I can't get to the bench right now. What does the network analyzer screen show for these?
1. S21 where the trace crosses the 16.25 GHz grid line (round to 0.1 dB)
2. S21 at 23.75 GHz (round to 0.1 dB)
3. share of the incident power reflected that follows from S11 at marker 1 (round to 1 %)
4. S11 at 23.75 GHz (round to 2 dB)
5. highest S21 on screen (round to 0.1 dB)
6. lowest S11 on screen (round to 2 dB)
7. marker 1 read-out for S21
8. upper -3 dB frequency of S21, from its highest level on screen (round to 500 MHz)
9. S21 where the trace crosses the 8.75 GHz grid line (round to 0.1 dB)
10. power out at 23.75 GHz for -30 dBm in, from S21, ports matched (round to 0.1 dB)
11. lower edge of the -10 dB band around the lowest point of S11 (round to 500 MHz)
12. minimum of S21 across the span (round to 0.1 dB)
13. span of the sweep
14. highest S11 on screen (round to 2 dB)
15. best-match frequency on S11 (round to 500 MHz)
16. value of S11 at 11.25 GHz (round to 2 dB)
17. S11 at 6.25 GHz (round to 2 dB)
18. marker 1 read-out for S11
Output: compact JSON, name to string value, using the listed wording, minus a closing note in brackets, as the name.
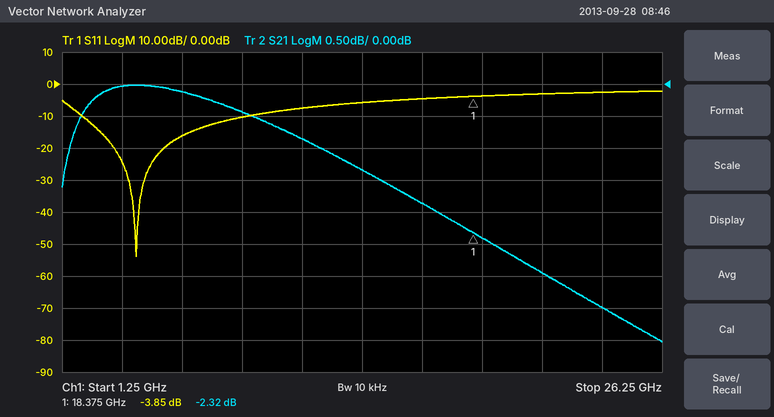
{"S21 where the trace crosses the 16.25 GHz grid line": "-1.9 dB", "S21 at 23.75 GHz": "-3.5 dB", "share of the incident power reflected that follows from S11 at marker 1": "41 %", "S11 at 23.75 GHz": "-2 dB", "highest S21 on screen": "0.0 dB", "lowest S11 on screen": "-54 dB", "marker 1 read-out for S21": "-2.32 dB", "upper -3 dB frequency of S21, from its highest level on screen": "21.5 GHz", "S21 where the trace crosses the 8.75 GHz grid line": "-0.4 dB", "power out at 23.75 GHz for -30 dBm in, from S21, ports matched": "-33.5 dBm", "lower edge of the -10 dB band around the lowest point of S11": "2.0 GHz", "minimum of S21 across the span": "-4.0 dB", "span of the sweep": "25 GHz", "highest S11 on screen": "-2 dB", "best-match frequency on S11": "4.5 GHz", "value of S11 at 11.25 GHz": "-8 dB", "S11 at 6.25 GHz": "-16 dB", "marker 1 read-out for S11": "-3.85 dB"}
